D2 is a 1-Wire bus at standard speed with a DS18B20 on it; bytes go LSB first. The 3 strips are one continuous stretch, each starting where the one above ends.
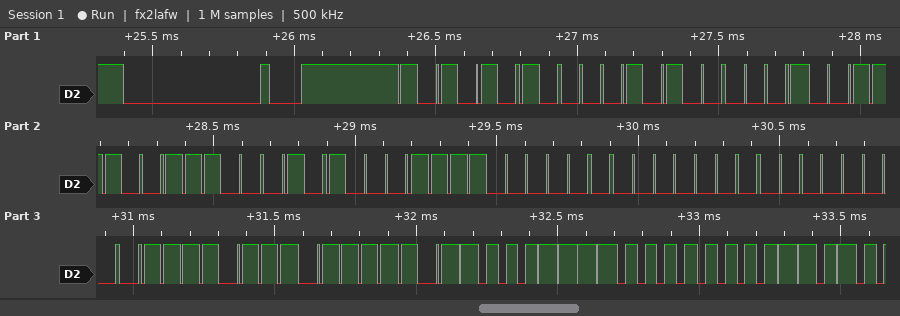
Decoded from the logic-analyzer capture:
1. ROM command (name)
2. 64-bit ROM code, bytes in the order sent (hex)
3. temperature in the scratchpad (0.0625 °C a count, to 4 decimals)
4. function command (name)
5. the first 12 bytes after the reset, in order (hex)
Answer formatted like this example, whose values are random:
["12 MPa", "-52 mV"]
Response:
["Match ROM", "28 C8 39 8A 07 00 00 EF", "15.0625 °C", "Read Scratchpad", "55 28 C8 39 8A 07 00 00 EF BE F1 00"]
